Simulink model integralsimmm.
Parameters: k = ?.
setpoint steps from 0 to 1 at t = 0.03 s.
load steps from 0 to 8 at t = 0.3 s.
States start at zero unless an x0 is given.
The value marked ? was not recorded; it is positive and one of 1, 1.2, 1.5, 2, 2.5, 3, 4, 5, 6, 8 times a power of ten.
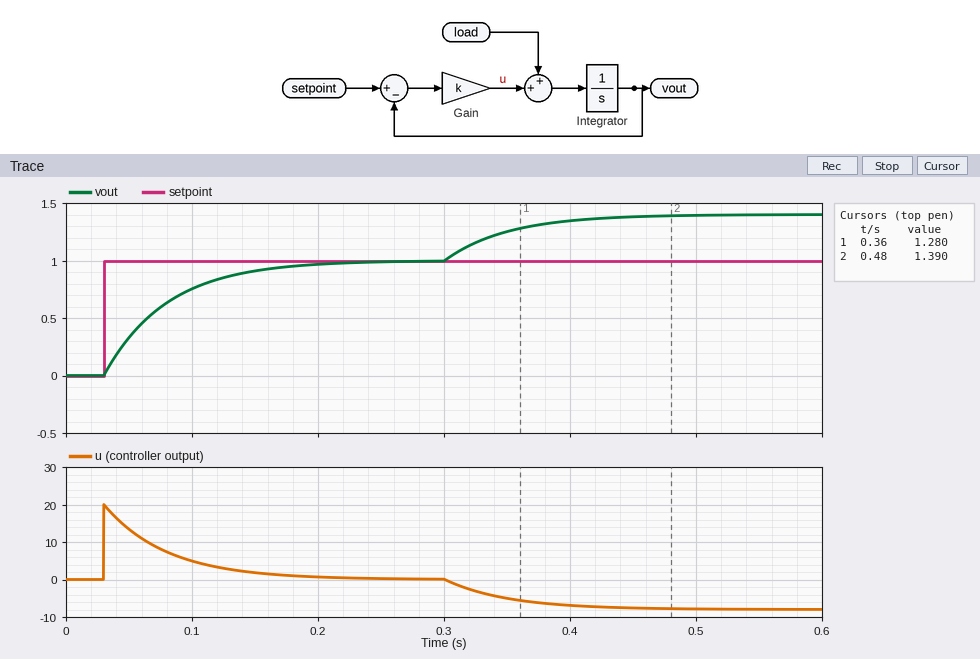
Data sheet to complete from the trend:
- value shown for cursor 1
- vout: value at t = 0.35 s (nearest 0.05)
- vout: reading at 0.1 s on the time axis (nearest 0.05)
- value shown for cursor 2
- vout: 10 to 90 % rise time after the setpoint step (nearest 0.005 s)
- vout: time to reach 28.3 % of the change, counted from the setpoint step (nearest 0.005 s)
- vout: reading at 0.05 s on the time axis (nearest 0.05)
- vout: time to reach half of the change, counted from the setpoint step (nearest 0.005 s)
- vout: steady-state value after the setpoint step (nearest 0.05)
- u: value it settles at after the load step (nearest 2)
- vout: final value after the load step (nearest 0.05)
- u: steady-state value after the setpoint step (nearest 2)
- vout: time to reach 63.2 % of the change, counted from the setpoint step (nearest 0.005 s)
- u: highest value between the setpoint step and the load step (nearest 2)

1.280
1.25
0.75
1.390
0.110 s
0.015 s
0.35
0.035 s
1.00
-8
1.40
0
0.050 s
20
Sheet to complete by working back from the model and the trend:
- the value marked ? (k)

20
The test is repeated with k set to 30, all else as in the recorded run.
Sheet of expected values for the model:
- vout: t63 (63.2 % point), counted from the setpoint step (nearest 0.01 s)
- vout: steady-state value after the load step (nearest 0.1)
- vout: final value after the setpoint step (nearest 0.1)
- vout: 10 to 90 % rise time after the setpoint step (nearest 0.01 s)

0.03 s
1.3
1.0
0.07 s
